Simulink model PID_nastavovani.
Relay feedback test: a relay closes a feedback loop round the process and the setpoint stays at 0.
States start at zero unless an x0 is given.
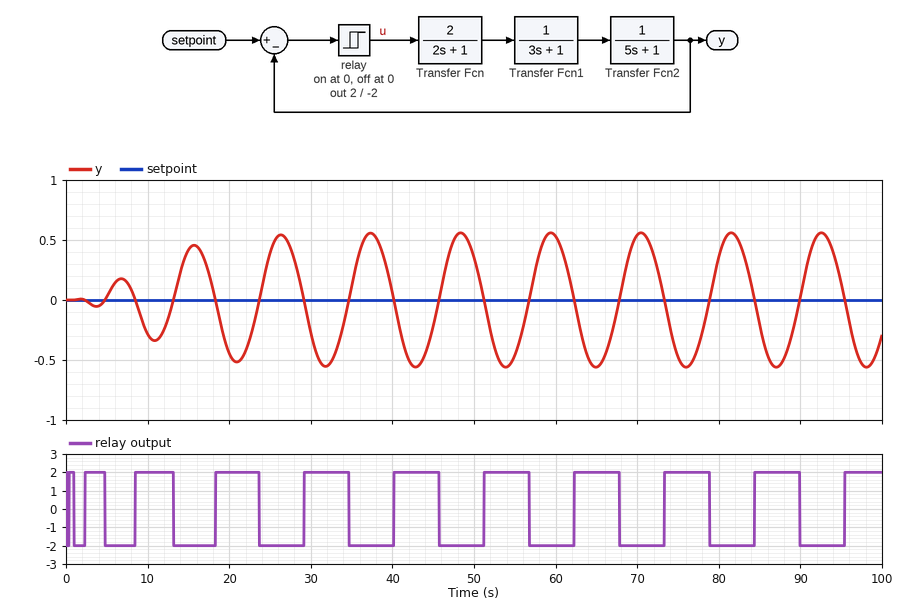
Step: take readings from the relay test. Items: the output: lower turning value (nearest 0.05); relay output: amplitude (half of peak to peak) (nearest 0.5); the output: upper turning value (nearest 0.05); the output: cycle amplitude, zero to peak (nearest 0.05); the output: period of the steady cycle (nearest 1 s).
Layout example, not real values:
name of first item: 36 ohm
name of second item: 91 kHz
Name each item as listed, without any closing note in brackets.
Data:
the output: lower turning value: -0.55
relay output: amplitude (half of peak to peak): 2.0
the output: upper turning value: 0.55
the output: cycle amplitude, zero to peak: 0.55
the output: period of the steady cycle: 11 s
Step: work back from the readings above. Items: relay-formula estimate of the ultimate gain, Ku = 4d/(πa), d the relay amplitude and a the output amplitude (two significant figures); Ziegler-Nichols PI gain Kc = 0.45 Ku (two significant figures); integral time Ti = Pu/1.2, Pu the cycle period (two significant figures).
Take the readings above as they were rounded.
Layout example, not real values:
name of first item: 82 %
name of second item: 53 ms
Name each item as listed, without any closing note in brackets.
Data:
relay-formula estimate of the ultimate gain, Ku = 4d/(πa), d the relay amplitude and a the output amplitude: 4.6
Ziegler-Nichols PI gain Kc = 0.45 Ku: 2.1
integral time Ti = Pu/1.2, Pu the cycle period: 9.2 s
